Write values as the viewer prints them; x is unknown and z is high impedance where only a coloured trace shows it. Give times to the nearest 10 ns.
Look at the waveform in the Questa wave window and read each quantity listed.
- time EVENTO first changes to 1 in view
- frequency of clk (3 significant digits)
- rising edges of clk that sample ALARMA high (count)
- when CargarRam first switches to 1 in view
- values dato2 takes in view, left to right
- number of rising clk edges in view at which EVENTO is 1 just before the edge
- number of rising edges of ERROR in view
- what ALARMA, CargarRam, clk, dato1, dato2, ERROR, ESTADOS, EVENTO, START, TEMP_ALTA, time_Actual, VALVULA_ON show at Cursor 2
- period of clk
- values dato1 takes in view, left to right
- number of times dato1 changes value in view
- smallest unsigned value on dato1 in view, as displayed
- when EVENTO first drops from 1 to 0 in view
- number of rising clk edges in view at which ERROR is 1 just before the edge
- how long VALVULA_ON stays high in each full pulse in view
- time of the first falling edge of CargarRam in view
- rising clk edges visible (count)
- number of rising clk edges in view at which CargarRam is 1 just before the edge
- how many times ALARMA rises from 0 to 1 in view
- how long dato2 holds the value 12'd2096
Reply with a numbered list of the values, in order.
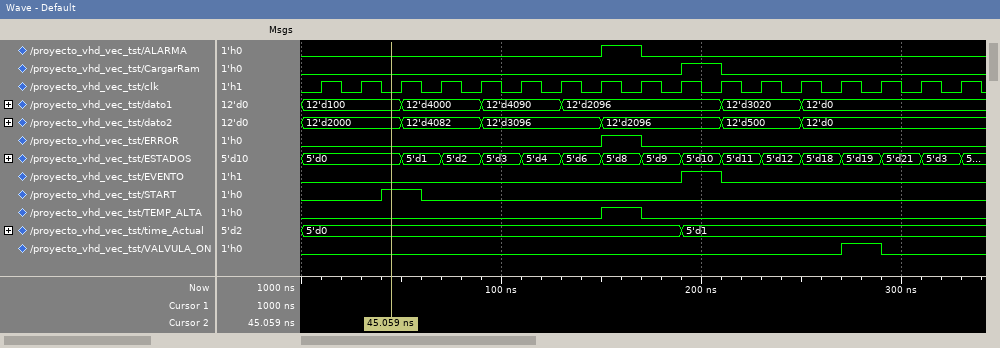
1. 190 ns
2. 50.0 MHz
3. 1
4. 190 ns
5. 12'd2000, 12'd4082, 12'd3096, 12'd2096, 12'd500, 12'd0
6. 1
7. 1
8. ALARMA=0, CargarRam=0, clk=0, dato1=12'd100, dato2=12'd2000, ERROR=0, ESTADOS=5'd0, EVENTO=0, START=1, TEMP_ALTA=0, time_Actual=5'd0, VALVULA_ON=0
9. 20 ns
10. 12'd100, 12'd4000, 12'd4090, 12'd2096, 12'd3020, 12'd0
11. 5
12. 12'd0
13. 210 ns
14. 1
15. 20 ns
16. 210 ns
17. 17
18. 1
19. 1
20. 60 ns
